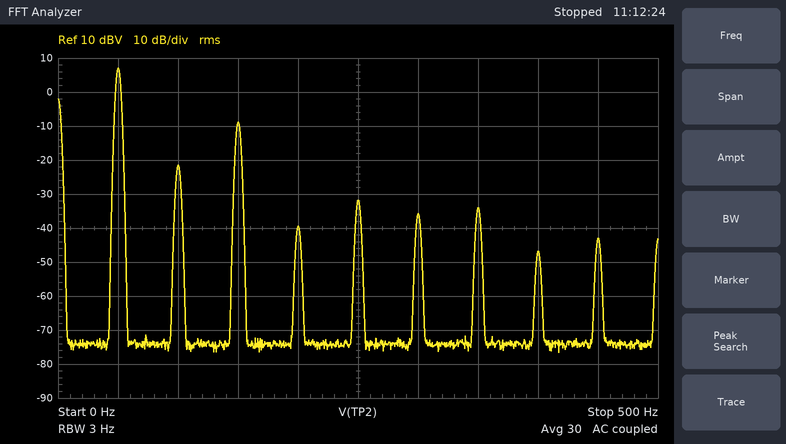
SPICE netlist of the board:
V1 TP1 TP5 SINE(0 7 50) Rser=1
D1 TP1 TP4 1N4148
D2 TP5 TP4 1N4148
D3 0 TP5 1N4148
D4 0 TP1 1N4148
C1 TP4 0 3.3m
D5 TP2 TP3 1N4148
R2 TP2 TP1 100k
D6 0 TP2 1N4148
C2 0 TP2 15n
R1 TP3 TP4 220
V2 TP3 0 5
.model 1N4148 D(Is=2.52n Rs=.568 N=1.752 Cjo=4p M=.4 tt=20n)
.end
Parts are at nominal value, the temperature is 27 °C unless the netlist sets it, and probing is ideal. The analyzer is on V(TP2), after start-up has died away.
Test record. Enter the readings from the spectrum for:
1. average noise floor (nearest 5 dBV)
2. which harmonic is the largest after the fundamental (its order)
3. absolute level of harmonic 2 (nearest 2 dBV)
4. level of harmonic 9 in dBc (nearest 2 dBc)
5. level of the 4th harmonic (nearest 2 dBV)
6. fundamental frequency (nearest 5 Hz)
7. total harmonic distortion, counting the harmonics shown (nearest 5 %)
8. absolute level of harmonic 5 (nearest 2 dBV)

-75 dBV
3
-22 dBV
-50 dBc
-40 dBV
50 Hz
15 %
-32 dBV
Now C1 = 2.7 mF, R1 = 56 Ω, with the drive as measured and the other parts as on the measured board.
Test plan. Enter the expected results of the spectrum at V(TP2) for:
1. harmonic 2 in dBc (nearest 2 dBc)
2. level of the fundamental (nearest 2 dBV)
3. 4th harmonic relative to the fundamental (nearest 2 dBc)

-32 dBc
8 dBV
-48 dBc
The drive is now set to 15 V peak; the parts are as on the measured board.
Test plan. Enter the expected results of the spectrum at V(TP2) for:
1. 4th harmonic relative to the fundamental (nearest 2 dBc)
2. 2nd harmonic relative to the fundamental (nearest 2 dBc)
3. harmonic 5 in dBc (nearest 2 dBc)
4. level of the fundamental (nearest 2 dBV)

-16 dBc
-10 dBc
-28 dBc
8 dBV
